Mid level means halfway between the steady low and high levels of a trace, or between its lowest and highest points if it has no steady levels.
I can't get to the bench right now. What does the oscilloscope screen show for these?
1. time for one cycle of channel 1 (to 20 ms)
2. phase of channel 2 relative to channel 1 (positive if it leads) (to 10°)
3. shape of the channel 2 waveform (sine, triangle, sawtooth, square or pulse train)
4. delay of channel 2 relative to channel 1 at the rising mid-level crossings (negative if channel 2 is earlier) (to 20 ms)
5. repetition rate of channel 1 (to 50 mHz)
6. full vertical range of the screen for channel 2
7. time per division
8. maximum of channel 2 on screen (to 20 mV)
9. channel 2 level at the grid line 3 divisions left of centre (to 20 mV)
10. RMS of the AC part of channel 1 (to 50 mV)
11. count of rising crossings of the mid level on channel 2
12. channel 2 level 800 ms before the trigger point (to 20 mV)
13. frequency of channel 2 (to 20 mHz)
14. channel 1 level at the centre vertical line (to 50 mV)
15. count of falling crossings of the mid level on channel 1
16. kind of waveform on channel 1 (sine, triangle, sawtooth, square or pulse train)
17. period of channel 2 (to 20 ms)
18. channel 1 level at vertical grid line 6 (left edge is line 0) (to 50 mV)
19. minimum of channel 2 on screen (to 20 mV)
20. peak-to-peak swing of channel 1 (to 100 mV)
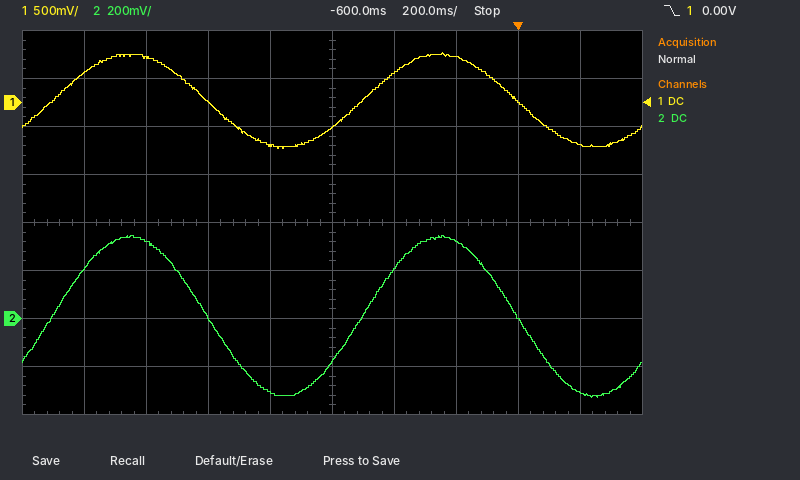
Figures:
1.00 s
0°
sine
0 ms
1.00 Hz
1.6 V
200 ms
340 mV
320 mV
350 mV
2
-300 mV
1.00 Hz
-250 mV
2
sine
1.00 s
300 mV
-320 mV
1.00 V
